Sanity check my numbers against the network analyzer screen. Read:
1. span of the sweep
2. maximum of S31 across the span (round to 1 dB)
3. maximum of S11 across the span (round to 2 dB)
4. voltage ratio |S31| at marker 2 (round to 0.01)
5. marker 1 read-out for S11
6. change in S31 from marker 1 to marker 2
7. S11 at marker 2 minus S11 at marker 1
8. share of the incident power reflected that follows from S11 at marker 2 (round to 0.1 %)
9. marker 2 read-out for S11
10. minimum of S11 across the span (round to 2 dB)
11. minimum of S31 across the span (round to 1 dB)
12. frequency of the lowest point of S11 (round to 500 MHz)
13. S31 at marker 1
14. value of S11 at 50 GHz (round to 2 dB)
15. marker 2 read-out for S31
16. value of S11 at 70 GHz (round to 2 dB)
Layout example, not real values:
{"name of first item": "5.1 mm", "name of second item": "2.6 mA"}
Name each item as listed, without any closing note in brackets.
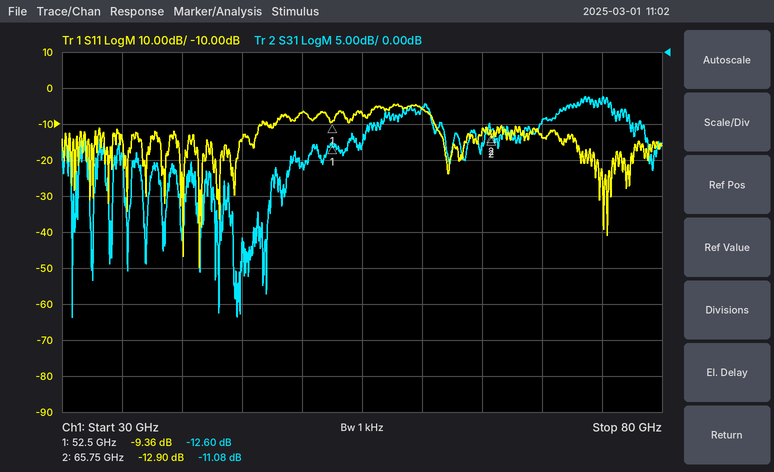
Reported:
{"span of the sweep": "50 GHz", "maximum of S31 across the span": "-6 dB", "maximum of S11 across the span": "-4 dB", "voltage ratio |S31| at marker 2": "0.28", "marker 1 read-out for S11": "-9.36 dB", "change in S31 from marker 1 to marker 2": "1.52 dB", "S11 at marker 2 minus S11 at marker 1": "-3.54 dB", "share of the incident power reflected that follows from S11 at marker 2": "5.1 %", "marker 2 read-out for S11": "-12.90 dB", "minimum of S11 across the span": "-50 dB", "minimum of S31 across the span": "-37 dB", "frequency of the lowest point of S11": "41.5 GHz", "S31 at marker 1": "-12.60 dB", "value of S11 at 50 GHz": "-6 dB", "marker 2 read-out for S31": "-11.08 dB", "value of S11 at 70 GHz": "-14 dB"}
